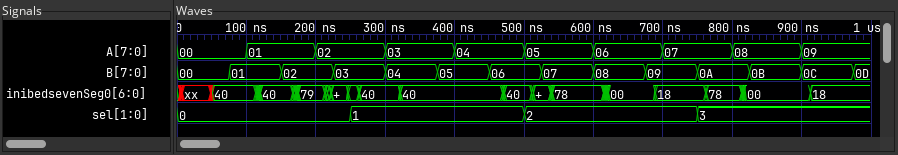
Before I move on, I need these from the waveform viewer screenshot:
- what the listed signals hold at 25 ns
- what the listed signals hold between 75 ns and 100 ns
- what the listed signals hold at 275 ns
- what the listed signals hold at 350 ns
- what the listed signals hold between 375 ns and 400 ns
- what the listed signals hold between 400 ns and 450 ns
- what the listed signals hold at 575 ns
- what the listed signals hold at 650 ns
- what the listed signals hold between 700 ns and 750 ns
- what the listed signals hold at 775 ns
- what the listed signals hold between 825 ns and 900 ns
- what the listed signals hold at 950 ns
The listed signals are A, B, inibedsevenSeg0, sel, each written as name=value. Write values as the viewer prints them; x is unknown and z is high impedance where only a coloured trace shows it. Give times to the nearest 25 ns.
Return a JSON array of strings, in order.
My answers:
["A=00, B=00, inibedsevenSeg0=xx, sel=0", "A=00, B=01, inibedsevenSeg0=40, sel=0", "A=02, B=03, inibedsevenSeg0=40, sel=1", "A=03, B=04, inibedsevenSeg0=40, sel=1", "A=03, B=05, inibedsevenSeg0=40, sel=1", "A=04, B=05, inibedsevenSeg0=40, sel=1", "A=05, B=07, inibedsevenSeg0=78, sel=2", "A=06, B=08, inibedsevenSeg0=00, sel=2", "A=07, B=09, inibedsevenSeg0=18, sel=2", "A=07, B=0A, inibedsevenSeg0=78, sel=3", "A=08, B=0B, inibedsevenSeg0=00, sel=3", "A=09, B=0C, inibedsevenSeg0=18, sel=3"]
